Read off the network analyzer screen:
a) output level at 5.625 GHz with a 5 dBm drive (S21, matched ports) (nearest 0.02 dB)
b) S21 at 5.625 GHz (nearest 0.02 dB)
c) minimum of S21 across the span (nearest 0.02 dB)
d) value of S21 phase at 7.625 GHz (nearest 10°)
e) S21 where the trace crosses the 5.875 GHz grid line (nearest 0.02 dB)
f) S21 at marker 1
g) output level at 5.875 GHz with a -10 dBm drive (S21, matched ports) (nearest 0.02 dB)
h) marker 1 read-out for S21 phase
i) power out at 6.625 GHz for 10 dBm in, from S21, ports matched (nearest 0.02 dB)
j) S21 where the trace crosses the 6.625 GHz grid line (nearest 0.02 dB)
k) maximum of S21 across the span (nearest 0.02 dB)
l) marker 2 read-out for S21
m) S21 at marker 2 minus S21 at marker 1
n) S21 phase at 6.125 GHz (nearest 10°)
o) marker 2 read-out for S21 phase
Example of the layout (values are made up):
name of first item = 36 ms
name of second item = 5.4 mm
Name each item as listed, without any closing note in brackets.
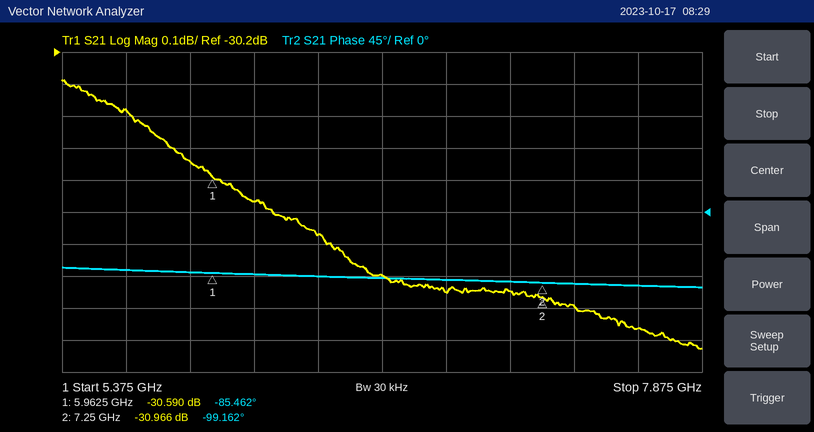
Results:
output level at 5.625 GHz with a 5 dBm drive (S21, matched ports) = -25.38 dBm
S21 at 5.625 GHz = -30.38 dB
minimum of S21 across the span = -31.12 dB
value of S21 phase at 7.625 GHz = -100°
S21 where the trace crosses the 5.875 GHz grid line = -30.54 dB
S21 at marker 1 = -30.590 dB
output level at 5.875 GHz with a -10 dBm drive (S21, matched ports) = -40.54 dBm
marker 1 read-out for S21 phase = -85.462°
power out at 6.625 GHz for 10 dBm in, from S21, ports matched = -20.90 dBm
S21 where the trace crosses the 6.625 GHz grid line = -30.90 dB
maximum of S21 across the span = -30.28 dB
marker 2 read-out for S21 = -30.966 dB
S21 at marker 2 minus S21 at marker 1 = -0.376 dB
S21 phase at 6.125 GHz = -90°
marker 2 read-out for S21 phase = -99.162°
